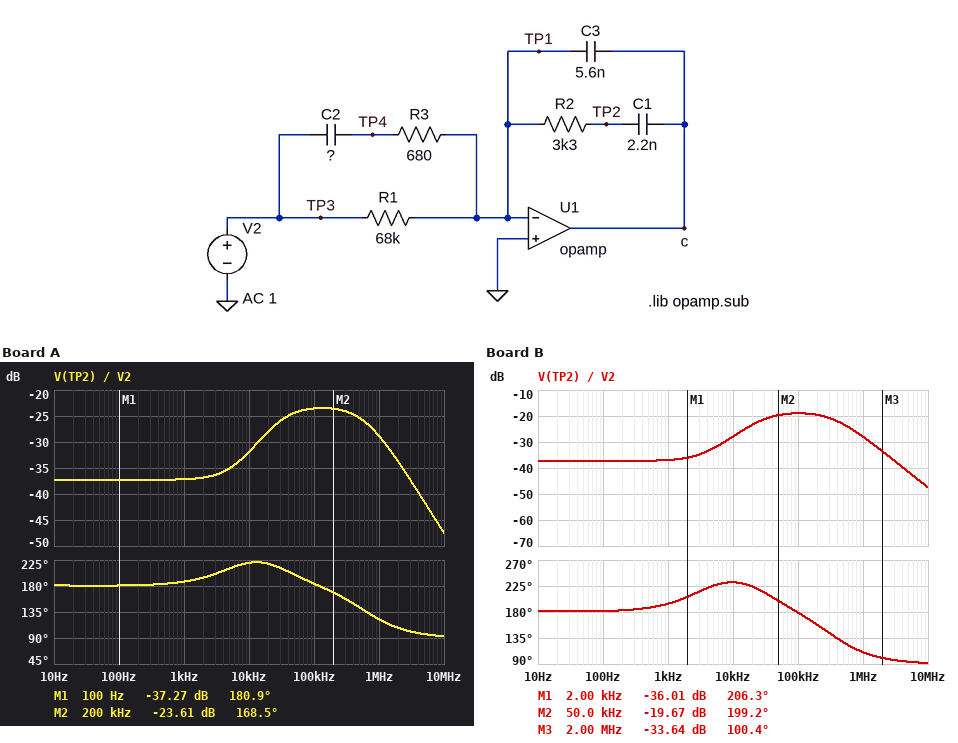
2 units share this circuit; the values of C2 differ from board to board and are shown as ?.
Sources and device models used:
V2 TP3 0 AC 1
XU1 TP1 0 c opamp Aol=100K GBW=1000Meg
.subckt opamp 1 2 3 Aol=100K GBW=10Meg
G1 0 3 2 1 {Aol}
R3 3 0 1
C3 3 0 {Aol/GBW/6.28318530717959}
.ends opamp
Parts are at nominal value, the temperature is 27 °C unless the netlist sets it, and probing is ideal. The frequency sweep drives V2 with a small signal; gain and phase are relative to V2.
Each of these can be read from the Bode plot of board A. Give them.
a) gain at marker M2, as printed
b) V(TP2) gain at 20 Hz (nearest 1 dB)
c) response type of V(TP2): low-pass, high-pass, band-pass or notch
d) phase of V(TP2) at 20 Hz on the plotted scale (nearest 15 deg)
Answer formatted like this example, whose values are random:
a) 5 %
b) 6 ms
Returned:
a) -23.61 dB
b) -37 dB
c) band-pass
d) 180 deg
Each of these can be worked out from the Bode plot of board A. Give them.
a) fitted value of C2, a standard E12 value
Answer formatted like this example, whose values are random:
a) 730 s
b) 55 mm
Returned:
a) 390 pF
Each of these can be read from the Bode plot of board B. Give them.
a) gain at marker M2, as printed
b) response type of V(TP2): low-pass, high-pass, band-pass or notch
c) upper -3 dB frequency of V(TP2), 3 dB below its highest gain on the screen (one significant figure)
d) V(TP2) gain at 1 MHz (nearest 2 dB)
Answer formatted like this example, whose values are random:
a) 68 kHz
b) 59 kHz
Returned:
a) -19.67 dB
b) band-pass
c) 400 kHz
d) -28 dB
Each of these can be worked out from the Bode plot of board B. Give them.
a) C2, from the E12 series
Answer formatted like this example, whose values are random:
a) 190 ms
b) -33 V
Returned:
a) 680 pF
